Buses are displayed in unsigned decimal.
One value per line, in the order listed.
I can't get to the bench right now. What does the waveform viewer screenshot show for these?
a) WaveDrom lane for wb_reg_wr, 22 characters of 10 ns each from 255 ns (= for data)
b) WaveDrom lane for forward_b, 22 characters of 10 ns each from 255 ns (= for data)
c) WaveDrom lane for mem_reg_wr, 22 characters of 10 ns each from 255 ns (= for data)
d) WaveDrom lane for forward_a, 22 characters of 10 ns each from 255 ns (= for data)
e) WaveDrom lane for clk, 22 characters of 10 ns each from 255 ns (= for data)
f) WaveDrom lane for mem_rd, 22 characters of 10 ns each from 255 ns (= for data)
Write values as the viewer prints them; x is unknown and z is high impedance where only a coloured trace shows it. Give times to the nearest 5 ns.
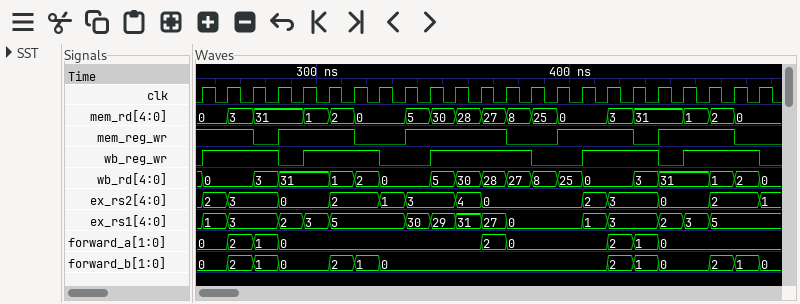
{name: 'wb_reg_wr', wave: '1..01..0.1...0.1..01..'}
{name: 'forward_b', wave: '====.===........===.==', data: '0 2 1 0 2 1 0 2 1 0 2 1'}
{name: 'mem_reg_wr', wave: '1.01..0.1...0.1..01..0'}
{name: 'forward_a', wave: '====.......==...===...', data: '0 2 1 0 2 0 2 1 0'}
{name: 'clk', wave: 'p.....................'}
{name: 'mem_rd', wave: '===.===.=======.==.===', data: '0 3 31 1 2 0 5 30 28 27 8 25 0 3 31 1 2 0'}
